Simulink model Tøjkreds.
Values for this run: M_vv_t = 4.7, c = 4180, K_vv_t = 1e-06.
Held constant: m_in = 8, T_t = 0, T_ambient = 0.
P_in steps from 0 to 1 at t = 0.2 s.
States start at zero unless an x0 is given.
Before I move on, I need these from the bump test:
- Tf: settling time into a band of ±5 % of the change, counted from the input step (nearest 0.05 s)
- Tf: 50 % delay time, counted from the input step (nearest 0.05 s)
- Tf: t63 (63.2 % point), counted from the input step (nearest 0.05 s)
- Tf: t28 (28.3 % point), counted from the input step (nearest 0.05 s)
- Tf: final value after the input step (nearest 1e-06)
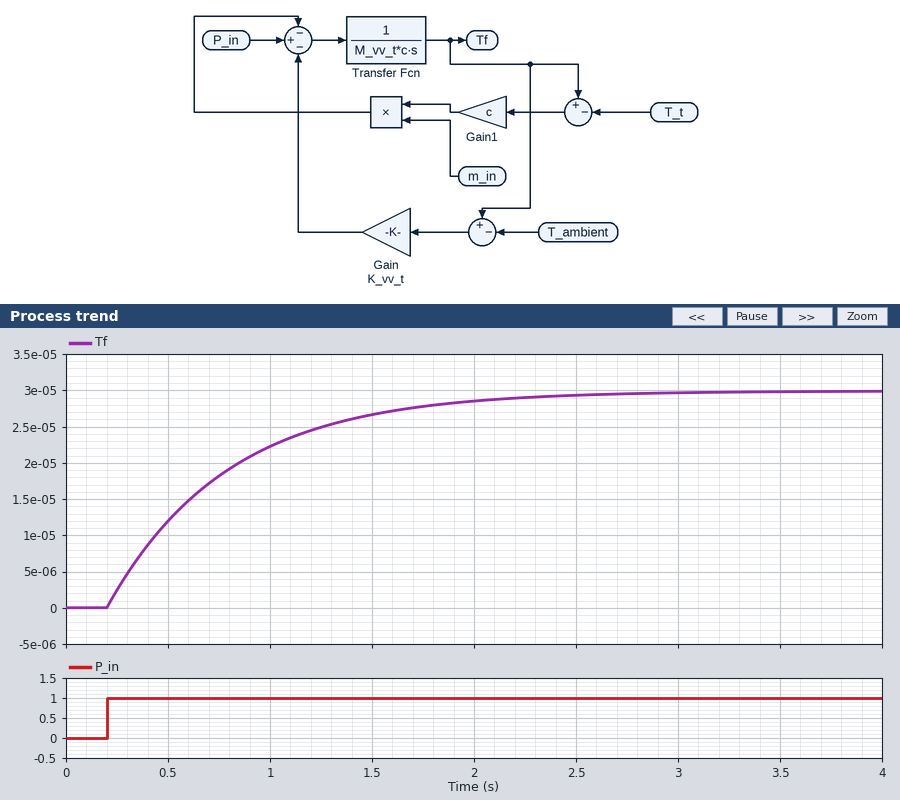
1.75 s
0.40 s
0.60 s
0.20 s
0.000030
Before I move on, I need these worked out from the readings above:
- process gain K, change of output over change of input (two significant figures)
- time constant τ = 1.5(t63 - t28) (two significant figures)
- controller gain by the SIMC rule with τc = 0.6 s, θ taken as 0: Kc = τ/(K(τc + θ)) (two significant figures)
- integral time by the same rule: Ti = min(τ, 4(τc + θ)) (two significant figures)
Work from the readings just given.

0.000030
0.60 s
33000
0.60 s
